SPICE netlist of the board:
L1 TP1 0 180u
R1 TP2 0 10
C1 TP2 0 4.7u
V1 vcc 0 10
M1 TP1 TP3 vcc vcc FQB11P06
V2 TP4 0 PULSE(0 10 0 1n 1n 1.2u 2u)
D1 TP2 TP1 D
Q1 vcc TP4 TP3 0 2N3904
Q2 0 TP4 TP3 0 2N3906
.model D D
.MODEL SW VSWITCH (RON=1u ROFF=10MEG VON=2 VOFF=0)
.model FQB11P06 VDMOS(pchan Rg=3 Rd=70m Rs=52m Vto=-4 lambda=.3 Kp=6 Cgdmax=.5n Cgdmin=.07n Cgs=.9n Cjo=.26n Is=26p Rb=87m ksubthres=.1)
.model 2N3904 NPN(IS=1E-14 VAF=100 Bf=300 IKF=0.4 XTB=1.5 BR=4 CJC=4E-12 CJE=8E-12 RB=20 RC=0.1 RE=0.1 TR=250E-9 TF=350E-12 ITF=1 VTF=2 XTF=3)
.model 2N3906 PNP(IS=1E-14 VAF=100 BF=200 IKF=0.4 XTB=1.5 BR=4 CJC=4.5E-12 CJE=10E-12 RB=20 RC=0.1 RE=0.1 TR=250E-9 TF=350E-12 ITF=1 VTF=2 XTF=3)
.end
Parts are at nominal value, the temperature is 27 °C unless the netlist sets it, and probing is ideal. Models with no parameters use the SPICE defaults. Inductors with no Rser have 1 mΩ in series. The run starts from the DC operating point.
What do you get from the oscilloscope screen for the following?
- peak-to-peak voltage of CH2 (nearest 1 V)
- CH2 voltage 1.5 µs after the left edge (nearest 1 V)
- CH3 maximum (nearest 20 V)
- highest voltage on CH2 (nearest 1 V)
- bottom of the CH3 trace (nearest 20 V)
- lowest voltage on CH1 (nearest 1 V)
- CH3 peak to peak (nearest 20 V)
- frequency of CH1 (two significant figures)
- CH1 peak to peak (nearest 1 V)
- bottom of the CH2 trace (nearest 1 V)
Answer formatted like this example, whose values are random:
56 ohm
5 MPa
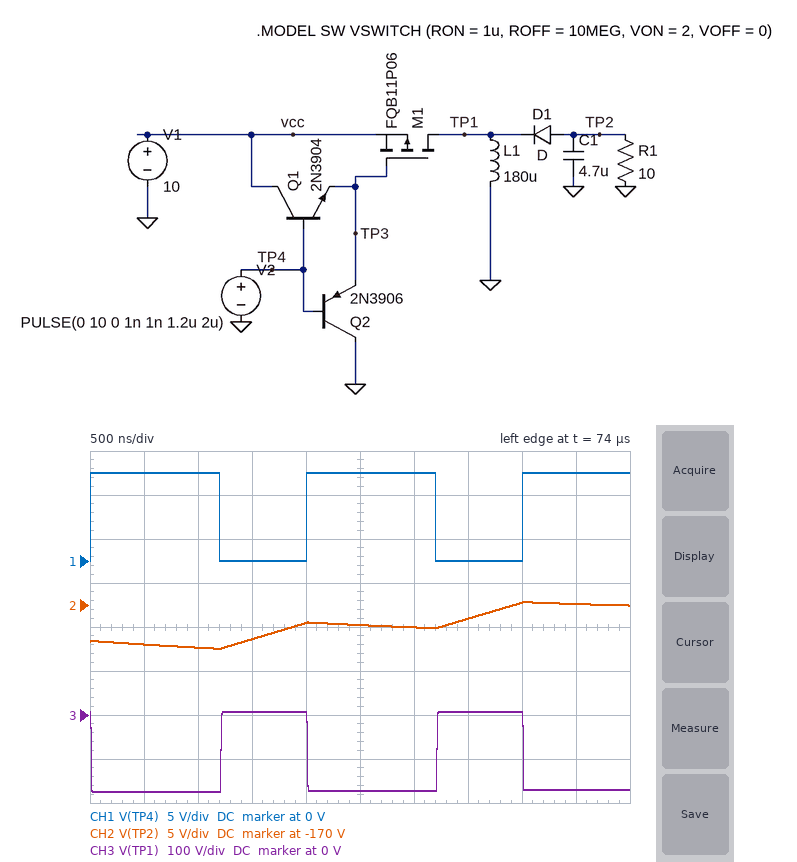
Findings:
5 V
-174 V
0 V
-170 V
-180 V
0 V
180 V
500 kHz
10 V
-175 V
